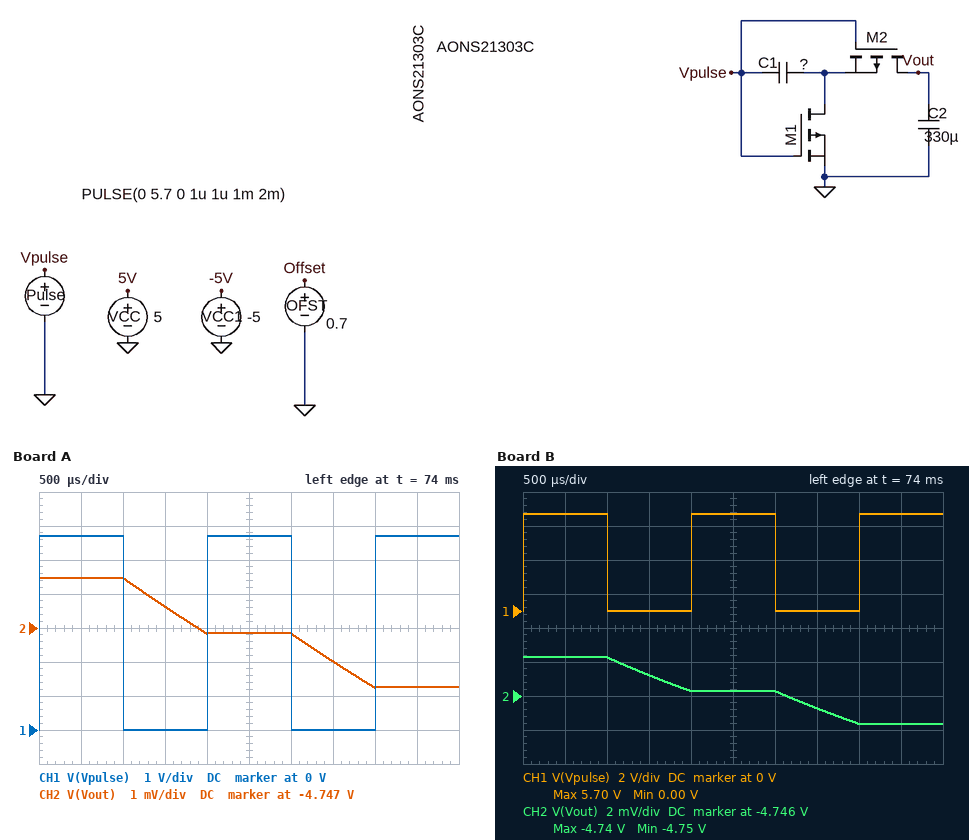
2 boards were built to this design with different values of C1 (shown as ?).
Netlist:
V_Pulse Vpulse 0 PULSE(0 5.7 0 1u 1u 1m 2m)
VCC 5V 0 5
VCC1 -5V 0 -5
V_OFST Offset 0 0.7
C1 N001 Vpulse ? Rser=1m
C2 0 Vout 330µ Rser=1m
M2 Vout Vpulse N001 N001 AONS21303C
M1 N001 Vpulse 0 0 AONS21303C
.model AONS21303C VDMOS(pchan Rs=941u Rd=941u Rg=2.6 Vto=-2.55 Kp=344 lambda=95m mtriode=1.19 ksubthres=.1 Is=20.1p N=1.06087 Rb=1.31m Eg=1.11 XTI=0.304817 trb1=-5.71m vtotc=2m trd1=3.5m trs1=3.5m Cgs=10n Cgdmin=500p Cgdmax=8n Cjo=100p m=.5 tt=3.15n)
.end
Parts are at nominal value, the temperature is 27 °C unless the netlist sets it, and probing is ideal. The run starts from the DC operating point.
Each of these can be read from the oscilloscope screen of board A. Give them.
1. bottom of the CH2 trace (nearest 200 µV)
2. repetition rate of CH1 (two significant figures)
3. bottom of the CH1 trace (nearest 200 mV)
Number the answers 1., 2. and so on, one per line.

1. -4.7488 V
2. 500 Hz
3. 0 V
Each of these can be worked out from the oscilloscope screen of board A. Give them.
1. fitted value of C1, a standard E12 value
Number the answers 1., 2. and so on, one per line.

1. 470 µF
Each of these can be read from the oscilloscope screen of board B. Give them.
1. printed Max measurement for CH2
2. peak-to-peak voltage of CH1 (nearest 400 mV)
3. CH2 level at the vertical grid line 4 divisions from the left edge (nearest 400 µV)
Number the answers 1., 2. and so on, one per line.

1. -4.74 V
2. 5.6 V
3. -4.7456 V
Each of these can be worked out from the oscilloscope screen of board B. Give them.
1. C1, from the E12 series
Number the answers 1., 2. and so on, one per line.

1. 150 µF
